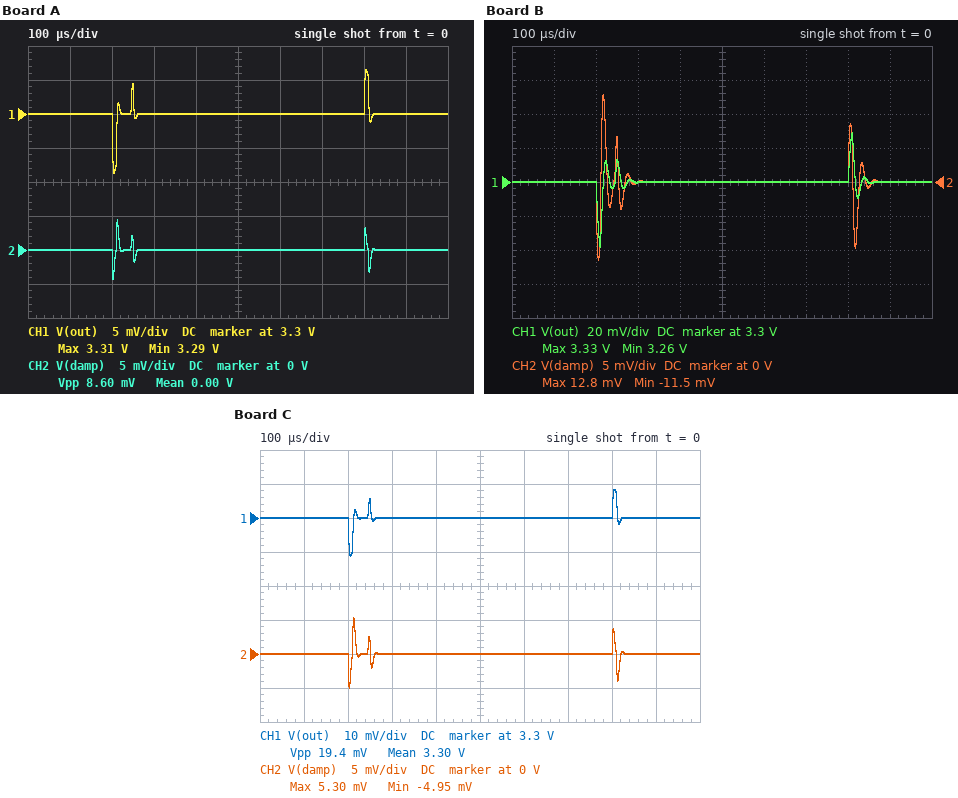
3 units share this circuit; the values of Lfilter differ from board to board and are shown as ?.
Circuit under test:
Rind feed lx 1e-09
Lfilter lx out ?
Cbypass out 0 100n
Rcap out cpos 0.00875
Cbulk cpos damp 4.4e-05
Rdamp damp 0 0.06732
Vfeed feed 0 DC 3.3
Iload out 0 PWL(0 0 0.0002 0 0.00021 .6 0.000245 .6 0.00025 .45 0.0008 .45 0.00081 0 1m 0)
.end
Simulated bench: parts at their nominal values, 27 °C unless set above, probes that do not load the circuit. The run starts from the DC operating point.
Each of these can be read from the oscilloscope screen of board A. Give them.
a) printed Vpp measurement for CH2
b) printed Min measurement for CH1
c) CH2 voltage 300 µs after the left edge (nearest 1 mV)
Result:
8.60 mV
3.29 V
0 V
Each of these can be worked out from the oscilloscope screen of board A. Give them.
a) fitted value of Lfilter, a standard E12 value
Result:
120 nH
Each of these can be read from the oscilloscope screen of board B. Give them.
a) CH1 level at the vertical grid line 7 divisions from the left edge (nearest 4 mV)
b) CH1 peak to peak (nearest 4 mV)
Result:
3.300 V
68 mV
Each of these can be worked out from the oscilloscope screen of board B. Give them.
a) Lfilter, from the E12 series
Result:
470 nH
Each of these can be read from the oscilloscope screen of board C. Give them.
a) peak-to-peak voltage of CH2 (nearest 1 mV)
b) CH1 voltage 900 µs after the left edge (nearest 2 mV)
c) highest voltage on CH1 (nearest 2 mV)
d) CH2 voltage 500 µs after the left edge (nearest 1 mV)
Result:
10 mV
3.300 V
3.308 V
0 V
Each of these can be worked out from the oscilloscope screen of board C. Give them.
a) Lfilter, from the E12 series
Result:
150 nH
